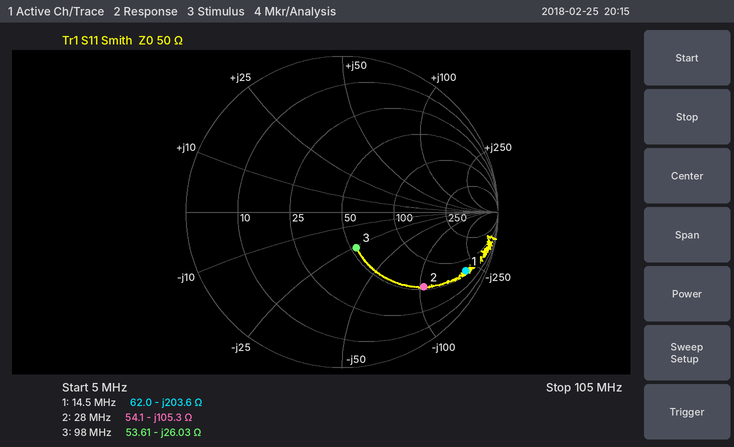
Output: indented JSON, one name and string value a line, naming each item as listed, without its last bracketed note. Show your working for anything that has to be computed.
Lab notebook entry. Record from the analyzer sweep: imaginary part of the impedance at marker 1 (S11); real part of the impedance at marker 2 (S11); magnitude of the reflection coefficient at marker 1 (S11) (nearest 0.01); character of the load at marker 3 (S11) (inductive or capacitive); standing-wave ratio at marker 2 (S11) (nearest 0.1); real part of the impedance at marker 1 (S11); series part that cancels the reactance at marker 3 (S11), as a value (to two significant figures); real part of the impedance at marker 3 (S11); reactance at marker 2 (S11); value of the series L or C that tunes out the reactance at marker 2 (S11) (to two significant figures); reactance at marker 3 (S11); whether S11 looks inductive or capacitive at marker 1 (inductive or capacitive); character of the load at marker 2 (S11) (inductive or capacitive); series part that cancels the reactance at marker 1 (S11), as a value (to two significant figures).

{
  "imaginary part of the impedance at marker 1": "-203.6 Ω",
  "real part of the impedance at marker 2": "54.1 Ω",
  "magnitude of the reflection coefficient at marker 1 (S11)": "0.88",
  "character of the load at marker 3 (S11)": "capacitive",
  "standing-wave ratio at marker 2 (S11)": "5.9",
  "real part of the impedance at marker 1": "62.0 Ω",
  "series part that cancels the reactance at marker 3 (S11), as a value": "L = 26.03 Ω/(2π × 98 MHz) ≈ 42 nH",
  "real part of the impedance at marker 3": "53.61 Ω",
  "reactance at marker 2": "-105.3 Ω",
  "value of the series L or C that tunes out the reactance at marker 2 (S11)": "L = 105.3 Ω/(2π × 28 MHz) ≈ 599 nH, so 600 nH to two significant figures",
  "reactance at marker 3": "-26.03 Ω",
  "whether S11 looks inductive or capacitive at marker 1": "capacitive",
  "character of the load at marker 2 (S11)": "capacitive",
  "series part that cancels the reactance at marker 1 (S11), as a value": "L = 203.6 Ω/(2π × 14.5 MHz) ≈ 2.2 µH"
}
